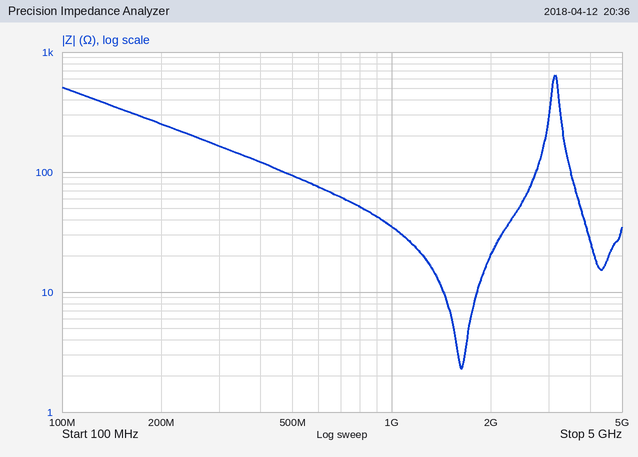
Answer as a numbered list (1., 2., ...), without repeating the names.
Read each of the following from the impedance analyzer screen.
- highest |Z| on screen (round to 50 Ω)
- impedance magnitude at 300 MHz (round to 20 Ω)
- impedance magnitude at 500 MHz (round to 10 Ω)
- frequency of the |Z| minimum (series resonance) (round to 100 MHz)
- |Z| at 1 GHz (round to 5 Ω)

1. 650 Ω
2. 160 Ω
3. 90 Ω
4. 1.6 GHz
5. 35 Ω
